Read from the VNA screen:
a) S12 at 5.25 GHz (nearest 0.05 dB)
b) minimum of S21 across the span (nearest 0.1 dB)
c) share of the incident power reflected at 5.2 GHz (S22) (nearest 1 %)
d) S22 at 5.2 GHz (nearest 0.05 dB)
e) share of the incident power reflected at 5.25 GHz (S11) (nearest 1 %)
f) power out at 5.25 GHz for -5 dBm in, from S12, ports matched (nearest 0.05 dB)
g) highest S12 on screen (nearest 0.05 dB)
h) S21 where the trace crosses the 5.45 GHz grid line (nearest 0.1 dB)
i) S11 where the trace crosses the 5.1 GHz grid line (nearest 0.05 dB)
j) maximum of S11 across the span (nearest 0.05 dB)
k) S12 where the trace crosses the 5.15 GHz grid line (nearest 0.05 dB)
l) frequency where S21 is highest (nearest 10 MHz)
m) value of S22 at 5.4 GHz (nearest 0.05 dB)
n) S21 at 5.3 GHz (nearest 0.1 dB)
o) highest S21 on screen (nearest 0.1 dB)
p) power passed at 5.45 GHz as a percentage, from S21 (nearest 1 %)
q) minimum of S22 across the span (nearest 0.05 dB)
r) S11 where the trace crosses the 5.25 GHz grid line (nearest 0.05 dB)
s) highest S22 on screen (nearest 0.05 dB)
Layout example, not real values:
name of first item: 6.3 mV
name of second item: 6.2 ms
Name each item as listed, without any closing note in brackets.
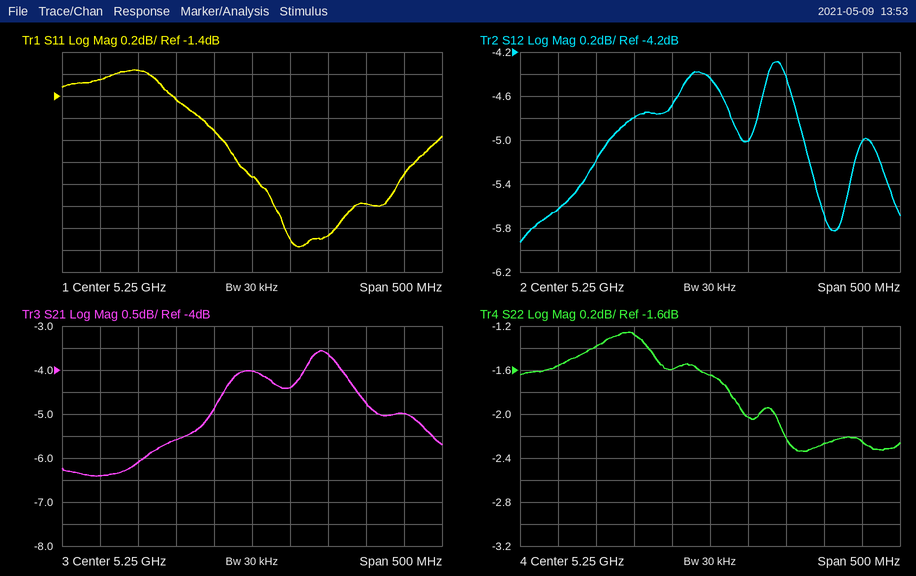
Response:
S12 at 5.25 GHz: -4.45 dB
minimum of S21 across the span: -6.4 dB
share of the incident power reflected at 5.2 GHz (S22): 69 %
S22 at 5.2 GHz: -1.60 dB
share of the incident power reflected at 5.25 GHz (S11): 61 %
power out at 5.25 GHz for -5 dBm in, from S12, ports matched: -9.45 dBm
highest S12 on screen: -4.30 dB
S21 where the trace crosses the 5.45 GHz grid line: -5.0 dB
S11 where the trace crosses the 5.1 GHz grid line: -1.15 dB
maximum of S11 across the span: -1.15 dB
S12 where the trace crosses the 5.15 GHz grid line: -4.80 dB
frequency where S21 is highest: 5.34 GHz
value of S22 at 5.4 GHz: -2.25 dB
S21 at 5.3 GHz: -4.4 dB
highest S21 on screen: -3.6 dB
power passed at 5.45 GHz as a percentage, from S21: 32 %
minimum of S22 across the span: -2.35 dB
S11 where the trace crosses the 5.25 GHz grid line: -2.15 dB
highest S22 on screen: -1.25 dB
